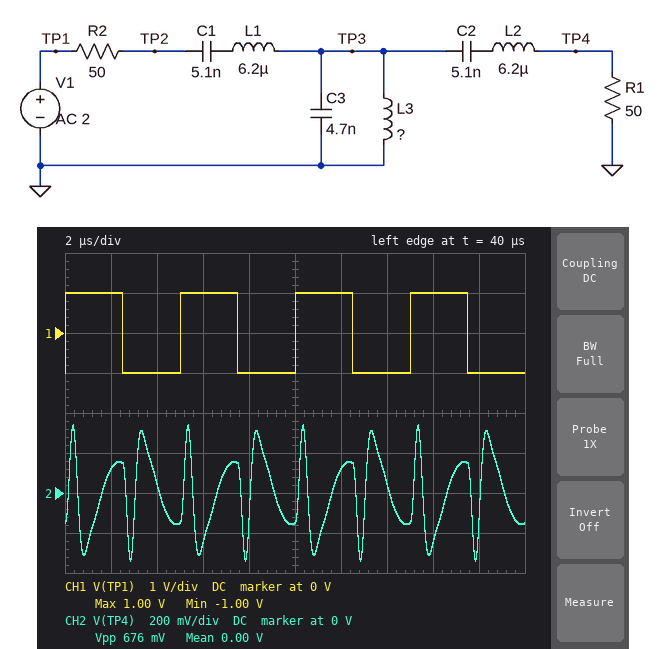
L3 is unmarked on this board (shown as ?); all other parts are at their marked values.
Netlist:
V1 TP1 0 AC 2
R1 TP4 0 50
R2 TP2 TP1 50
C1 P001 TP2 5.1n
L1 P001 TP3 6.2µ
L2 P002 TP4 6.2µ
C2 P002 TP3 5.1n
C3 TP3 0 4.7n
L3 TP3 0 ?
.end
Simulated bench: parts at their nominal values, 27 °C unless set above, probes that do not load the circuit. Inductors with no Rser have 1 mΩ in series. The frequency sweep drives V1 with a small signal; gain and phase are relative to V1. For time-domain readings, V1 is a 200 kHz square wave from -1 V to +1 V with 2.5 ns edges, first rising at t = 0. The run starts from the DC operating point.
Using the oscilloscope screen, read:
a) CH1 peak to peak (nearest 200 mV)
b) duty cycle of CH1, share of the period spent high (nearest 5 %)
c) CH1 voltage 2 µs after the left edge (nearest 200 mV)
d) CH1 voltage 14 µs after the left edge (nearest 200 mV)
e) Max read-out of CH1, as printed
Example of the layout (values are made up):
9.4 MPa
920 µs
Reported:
2.0 V
50 %
1.0 V
-1.0 V
1.00 V
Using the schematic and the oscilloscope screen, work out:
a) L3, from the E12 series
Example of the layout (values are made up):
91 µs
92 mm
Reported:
18 µH
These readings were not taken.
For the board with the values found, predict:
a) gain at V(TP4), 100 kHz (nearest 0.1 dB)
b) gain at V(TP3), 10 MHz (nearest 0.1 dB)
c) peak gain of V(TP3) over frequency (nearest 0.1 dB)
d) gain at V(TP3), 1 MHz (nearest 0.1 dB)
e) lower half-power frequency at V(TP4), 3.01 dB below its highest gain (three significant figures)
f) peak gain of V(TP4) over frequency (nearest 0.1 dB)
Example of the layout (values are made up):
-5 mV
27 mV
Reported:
-43.8 dB
-41.0 dB
-0.1 dB
-6.5 dB
278 kHz
-6.0 dB
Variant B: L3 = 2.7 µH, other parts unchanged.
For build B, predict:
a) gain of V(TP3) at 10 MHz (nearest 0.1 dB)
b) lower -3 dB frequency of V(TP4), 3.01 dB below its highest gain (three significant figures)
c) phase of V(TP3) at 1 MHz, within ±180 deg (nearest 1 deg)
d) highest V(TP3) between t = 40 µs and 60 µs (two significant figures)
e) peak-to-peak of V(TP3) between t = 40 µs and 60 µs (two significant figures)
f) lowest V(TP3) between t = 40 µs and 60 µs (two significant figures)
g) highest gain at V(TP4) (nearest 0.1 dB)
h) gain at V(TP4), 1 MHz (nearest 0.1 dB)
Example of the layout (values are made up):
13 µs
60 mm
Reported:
-40.9 dB
882 kHz
33 deg
440 mV
880 mV
-440 mV
-6.0 dB
-8.6 dB
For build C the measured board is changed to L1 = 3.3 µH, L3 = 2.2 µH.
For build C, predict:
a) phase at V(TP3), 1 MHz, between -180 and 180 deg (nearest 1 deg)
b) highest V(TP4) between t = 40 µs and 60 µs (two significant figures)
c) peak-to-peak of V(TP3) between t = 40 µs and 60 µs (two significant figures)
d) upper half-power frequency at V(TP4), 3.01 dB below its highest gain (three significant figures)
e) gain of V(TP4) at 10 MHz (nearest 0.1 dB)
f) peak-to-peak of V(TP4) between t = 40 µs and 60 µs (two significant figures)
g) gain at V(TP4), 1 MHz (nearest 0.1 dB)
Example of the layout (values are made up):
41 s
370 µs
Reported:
59 deg
330 mV
920 mV
2.31 MHz
-53.3 dB
660 mV
-9.4 dB
